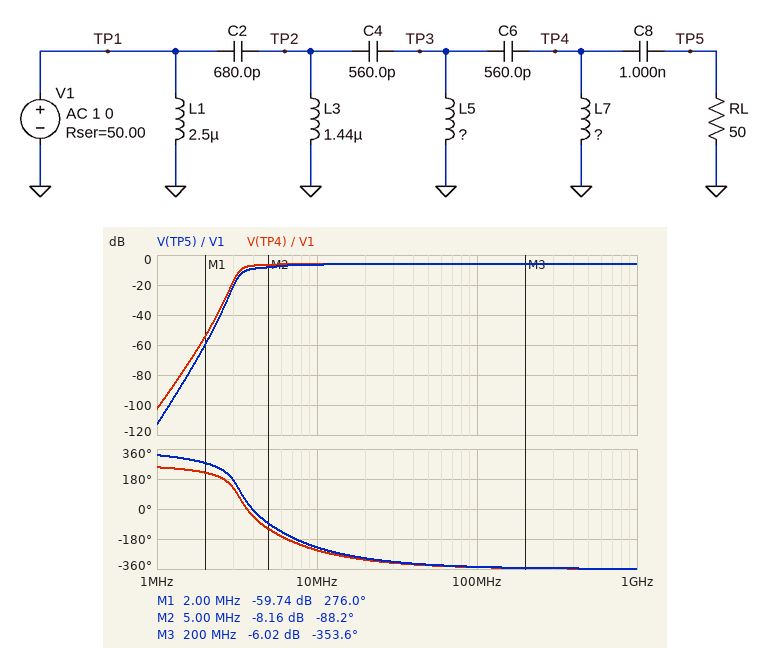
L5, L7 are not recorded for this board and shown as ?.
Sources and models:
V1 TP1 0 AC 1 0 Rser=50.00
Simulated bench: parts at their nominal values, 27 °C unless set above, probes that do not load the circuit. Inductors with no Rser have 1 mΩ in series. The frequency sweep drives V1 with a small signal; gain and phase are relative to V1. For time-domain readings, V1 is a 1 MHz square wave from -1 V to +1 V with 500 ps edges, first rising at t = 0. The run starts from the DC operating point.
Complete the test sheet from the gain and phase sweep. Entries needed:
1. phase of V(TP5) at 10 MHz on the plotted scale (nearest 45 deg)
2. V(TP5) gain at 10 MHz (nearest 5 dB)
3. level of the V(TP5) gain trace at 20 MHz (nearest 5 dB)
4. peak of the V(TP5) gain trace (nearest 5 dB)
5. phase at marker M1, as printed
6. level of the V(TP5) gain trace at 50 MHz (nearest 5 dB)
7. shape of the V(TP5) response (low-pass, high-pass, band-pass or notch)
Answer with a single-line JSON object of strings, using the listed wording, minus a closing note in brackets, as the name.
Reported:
{"phase of V(TP5) at 10 MHz on the plotted scale": "-225 deg", "V(TP5) gain at 10 MHz": "-5 dB", "level of the V(TP5) gain trace at 20 MHz": "-5 dB", "peak of the V(TP5) gain trace": "-5 dB", "phase at marker M1, as printed": "276.0 deg", "level of the V(TP5) gain trace at 50 MHz": "-5 dB", "shape of the V(TP5) response": "high-pass"}
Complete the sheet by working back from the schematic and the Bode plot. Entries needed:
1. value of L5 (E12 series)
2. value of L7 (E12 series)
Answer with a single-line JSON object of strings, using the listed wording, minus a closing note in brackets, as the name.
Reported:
{"value of L5": "680 nH", "value of L7": "1.5 µH"}
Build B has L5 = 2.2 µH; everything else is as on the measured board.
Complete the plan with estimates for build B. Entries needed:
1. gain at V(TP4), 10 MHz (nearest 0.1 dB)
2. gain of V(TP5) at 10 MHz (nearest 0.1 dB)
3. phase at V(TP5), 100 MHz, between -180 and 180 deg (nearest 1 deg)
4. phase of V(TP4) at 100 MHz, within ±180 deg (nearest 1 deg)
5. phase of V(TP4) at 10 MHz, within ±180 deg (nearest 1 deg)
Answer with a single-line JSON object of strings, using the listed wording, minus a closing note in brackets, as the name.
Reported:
{"gain at V(TP4), 10 MHz": "-5.7 dB", "gain of V(TP5) at 10 MHz": "-6.1 dB", "phase at V(TP5), 100 MHz, between -180 and 180 deg": "11 deg", "phase of V(TP4) at 100 MHz, within ±180 deg": "9 deg", "phase of V(TP4) at 10 MHz, within ±180 deg": "89 deg"}
